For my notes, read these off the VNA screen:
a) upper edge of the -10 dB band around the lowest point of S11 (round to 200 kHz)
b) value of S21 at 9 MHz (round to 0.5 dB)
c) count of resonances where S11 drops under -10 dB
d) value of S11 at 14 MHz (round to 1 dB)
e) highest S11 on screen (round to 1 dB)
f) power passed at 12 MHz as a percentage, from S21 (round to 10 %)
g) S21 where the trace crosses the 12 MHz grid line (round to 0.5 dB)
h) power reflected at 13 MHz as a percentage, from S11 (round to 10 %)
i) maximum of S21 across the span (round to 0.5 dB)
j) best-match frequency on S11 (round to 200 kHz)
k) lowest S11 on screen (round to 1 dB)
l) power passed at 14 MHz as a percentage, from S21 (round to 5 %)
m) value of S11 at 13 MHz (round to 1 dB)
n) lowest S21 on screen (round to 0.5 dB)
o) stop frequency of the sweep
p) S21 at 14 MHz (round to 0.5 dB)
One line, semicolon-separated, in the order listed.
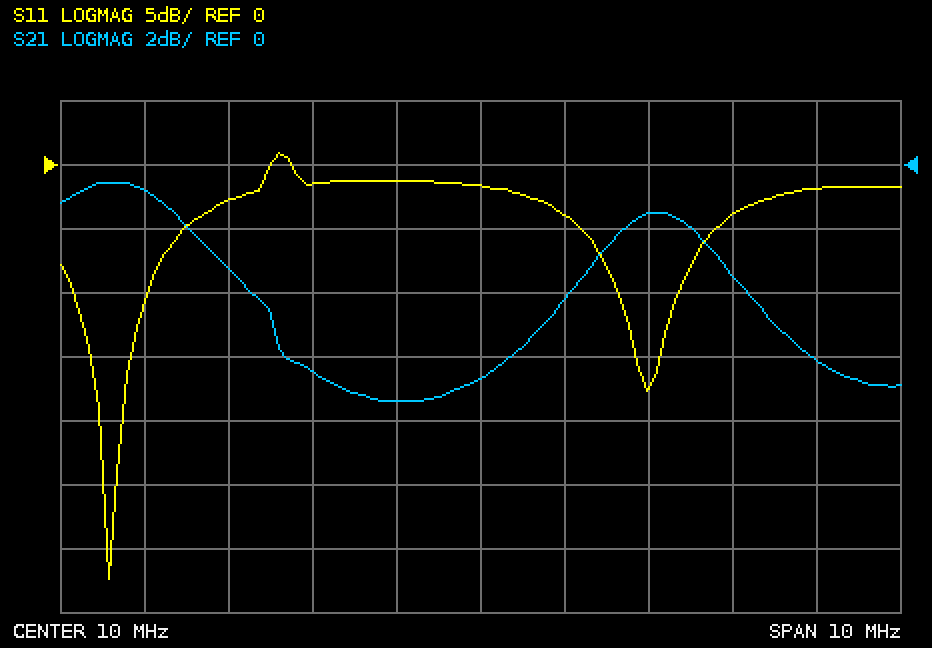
6.0 MHz; -7.5 dB; 2; -2 dB; 1 dB; 70 %; -1.5 dB; 40 %; -0.5 dB; 5.6 MHz; -32 dB; 25 %; -4 dB; -7.5 dB; 15 MHz; -6.0 dB
